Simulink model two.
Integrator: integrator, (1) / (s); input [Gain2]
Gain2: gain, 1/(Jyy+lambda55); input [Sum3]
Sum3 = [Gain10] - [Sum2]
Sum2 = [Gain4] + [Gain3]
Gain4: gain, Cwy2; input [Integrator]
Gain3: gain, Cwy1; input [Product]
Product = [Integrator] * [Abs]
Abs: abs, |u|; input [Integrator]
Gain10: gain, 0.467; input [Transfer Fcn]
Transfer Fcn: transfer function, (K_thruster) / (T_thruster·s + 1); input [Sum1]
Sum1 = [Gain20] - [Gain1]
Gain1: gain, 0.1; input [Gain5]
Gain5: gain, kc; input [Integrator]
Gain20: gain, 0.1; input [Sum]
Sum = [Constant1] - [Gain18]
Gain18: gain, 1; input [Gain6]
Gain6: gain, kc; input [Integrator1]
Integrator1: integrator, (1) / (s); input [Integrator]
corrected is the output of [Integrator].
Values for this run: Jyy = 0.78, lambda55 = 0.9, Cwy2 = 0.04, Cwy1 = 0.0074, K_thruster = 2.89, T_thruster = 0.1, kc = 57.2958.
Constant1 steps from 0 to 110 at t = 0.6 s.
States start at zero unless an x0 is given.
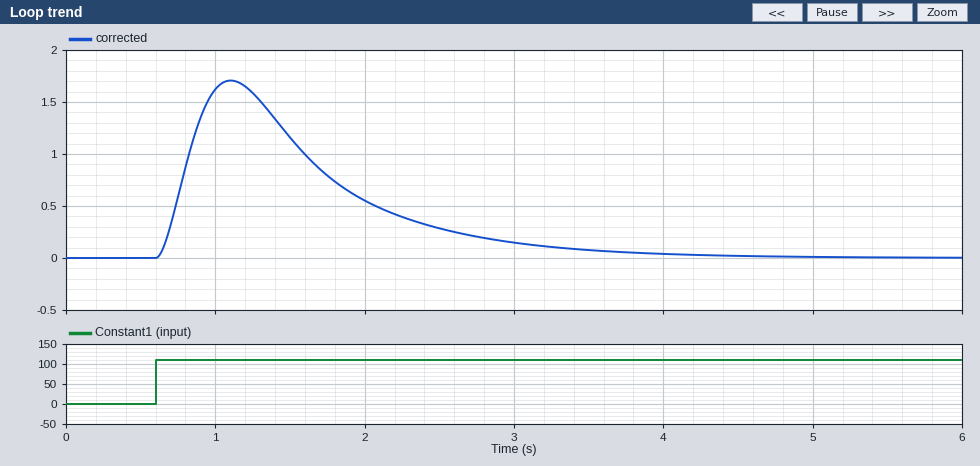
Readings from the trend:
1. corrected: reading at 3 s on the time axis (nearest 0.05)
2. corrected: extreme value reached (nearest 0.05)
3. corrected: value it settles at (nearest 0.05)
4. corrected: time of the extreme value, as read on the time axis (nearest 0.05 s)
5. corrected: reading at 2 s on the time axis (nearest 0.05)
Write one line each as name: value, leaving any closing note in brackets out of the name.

corrected: reading at 3 s on the time axis: 0.15
corrected: extreme value reached: 1.70
corrected: value it settles at: 0.00
corrected: time of the extreme value, as read on the time axis: 1.10 s
corrected: reading at 2 s on the time axis: 0.55
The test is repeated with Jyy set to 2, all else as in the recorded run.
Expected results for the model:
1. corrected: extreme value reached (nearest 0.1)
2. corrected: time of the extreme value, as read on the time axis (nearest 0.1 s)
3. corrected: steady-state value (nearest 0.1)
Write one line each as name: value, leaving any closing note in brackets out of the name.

corrected: extreme value reached: 1.5
corrected: time of the extreme value, as read on the time axis: 1.3 s
corrected: steady-state value: 0.0
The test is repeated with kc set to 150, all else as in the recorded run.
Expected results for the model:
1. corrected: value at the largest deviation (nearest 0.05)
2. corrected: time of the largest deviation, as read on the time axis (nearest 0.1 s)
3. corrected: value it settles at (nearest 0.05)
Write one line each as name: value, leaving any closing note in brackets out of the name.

corrected: value at the largest deviation: 0.80
corrected: time of the largest deviation, as read on the time axis: 0.9 s
corrected: value it settles at: 0.00
